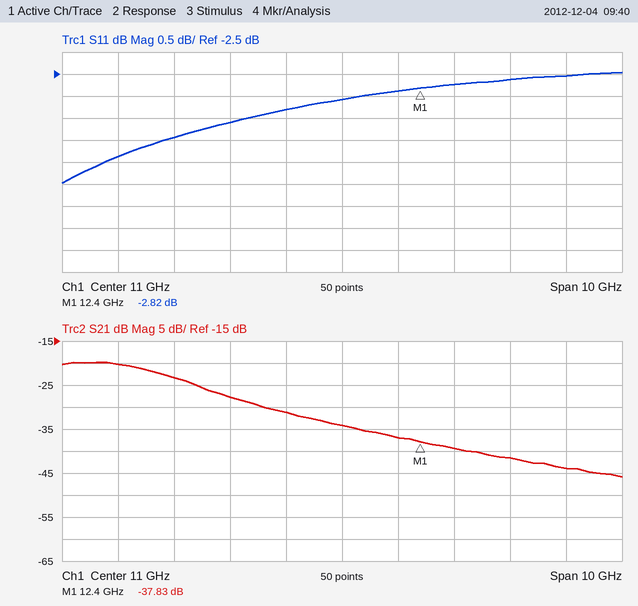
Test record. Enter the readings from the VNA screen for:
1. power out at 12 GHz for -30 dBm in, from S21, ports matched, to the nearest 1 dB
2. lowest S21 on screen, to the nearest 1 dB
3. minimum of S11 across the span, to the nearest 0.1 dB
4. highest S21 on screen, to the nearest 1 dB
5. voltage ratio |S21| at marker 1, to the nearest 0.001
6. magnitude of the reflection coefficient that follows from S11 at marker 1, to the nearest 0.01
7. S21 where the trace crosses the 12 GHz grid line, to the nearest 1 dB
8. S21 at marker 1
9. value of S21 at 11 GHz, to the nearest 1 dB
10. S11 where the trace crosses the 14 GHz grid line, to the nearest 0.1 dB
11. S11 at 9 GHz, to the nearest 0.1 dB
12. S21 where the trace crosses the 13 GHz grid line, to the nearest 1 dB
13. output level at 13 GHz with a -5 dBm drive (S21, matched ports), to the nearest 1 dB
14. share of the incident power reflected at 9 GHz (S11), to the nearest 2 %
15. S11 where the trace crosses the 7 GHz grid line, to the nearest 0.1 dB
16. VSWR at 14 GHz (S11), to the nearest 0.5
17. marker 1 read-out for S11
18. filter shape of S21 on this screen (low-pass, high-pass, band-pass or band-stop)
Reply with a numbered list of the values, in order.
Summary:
1. -67 dBm
2. -46 dB
3. -5.0 dB
4. -20 dB
5. 0.013
6. 0.72
7. -37 dB
8. -37.83 dB
9. -34 dB
10. -2.6 dB
11. -3.6 dB
12. -39 dB
13. -44 dBm
14. 44 %
15. -4.4 dB
16. 6.5
17. -2.82 dB
18. low-pass
